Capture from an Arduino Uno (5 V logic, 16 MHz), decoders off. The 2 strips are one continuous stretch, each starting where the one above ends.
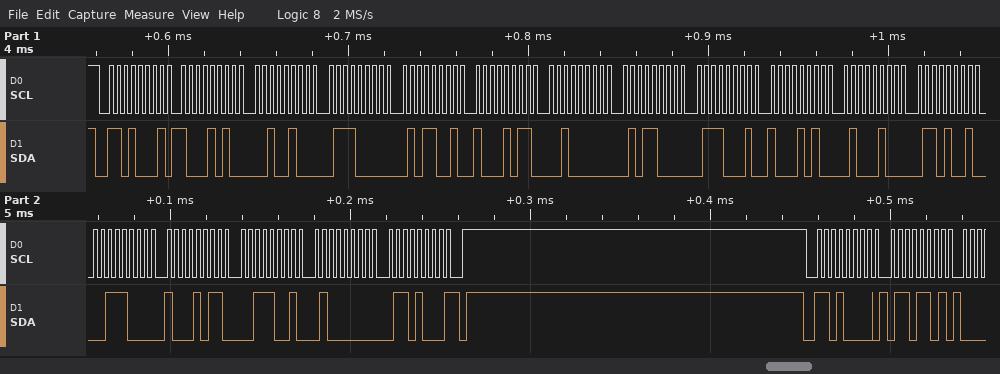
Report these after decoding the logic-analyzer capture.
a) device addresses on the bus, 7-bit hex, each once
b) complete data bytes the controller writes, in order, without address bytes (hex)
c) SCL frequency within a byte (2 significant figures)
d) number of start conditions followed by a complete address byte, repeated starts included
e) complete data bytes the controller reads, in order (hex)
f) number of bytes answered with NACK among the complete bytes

0x68
6D
250 kHz
2
8A 24 70 59 8B 20 58 71 8A 44 69 38 8B 39 40 68
1
